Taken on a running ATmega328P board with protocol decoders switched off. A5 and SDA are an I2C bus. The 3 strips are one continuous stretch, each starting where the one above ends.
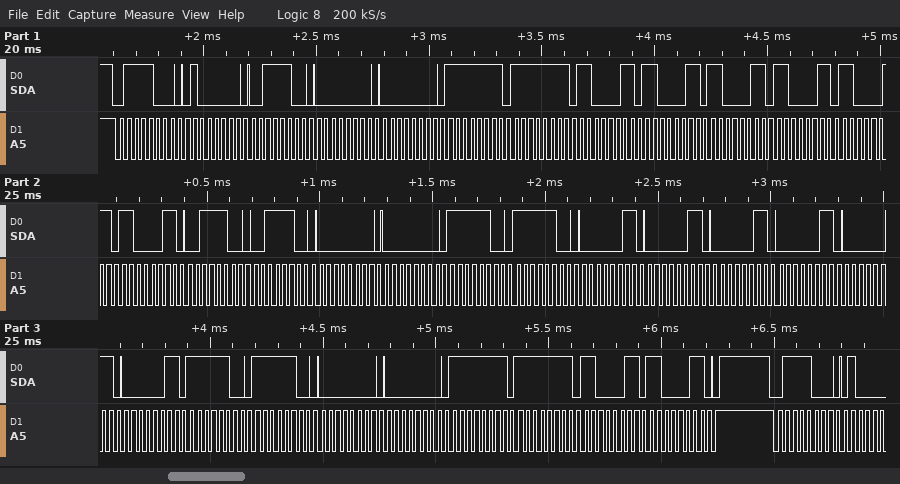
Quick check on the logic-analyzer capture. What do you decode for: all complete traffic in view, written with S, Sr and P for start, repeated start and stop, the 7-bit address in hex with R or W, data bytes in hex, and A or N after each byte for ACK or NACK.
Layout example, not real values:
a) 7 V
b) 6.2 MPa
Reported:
a) S 3CW A 40 A 3C A 00 A 00 A FF A FF A C3 A C3 A C3 A C3 A C3 A C3 A 3C A 3C A 00 A 00 A FC A FC A 03 A 03 A 03 A 03 A 03 A 03 A FC A FC A 00 A 00 A FF A FF A C3 A C3 A P S 3CW A
